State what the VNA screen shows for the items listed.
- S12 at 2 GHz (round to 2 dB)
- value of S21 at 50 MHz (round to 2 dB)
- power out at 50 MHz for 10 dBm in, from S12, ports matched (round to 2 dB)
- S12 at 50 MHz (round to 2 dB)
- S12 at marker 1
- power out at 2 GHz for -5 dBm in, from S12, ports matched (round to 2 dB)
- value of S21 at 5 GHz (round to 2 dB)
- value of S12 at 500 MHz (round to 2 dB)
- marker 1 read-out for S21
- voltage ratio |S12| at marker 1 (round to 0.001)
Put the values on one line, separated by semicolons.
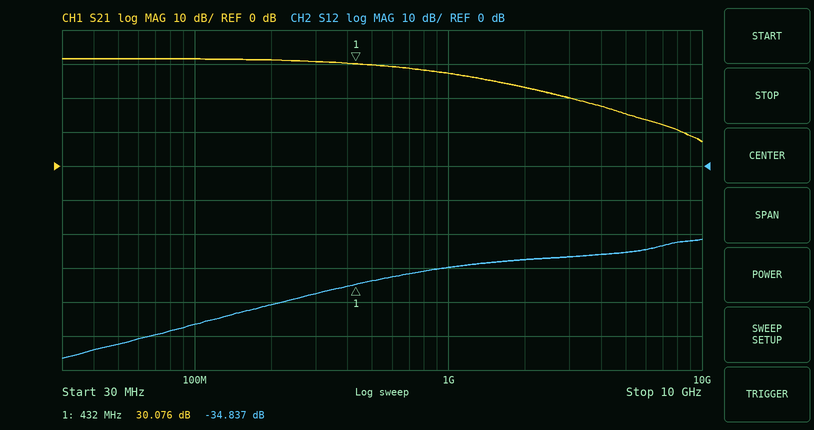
-28 dB; 32 dB; -42 dBm; -52 dB; -34.837 dB; -32 dBm; 16 dB; -34 dB; 30.076 dB; 0.018
